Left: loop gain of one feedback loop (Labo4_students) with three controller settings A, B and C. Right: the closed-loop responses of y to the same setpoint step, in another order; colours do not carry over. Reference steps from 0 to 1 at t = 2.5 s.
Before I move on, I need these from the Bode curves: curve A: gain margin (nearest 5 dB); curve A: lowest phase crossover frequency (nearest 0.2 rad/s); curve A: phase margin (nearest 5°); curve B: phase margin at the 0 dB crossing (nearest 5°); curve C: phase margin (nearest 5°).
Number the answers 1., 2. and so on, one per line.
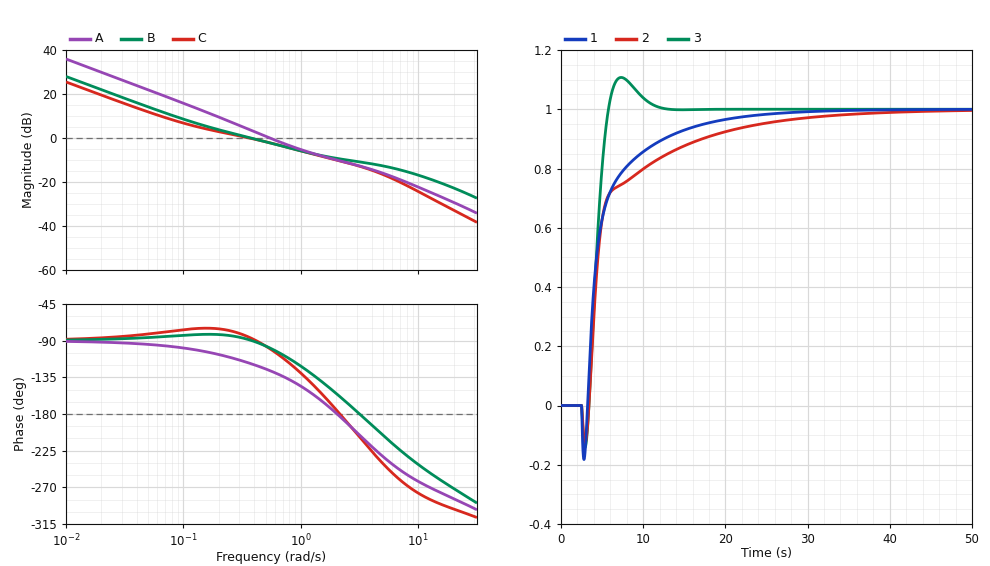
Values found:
1. 10 dB
2. 2.0 rad/s
3. 55°
4. 90°
5. 95°
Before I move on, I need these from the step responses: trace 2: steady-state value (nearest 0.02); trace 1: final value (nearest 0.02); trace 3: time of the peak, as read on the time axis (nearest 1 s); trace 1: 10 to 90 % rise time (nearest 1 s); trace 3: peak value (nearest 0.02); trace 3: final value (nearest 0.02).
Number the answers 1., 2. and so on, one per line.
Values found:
1. 1.00
2. 1.00
3. 7 s
4. 9 s
5. 1.10
6. 1.00
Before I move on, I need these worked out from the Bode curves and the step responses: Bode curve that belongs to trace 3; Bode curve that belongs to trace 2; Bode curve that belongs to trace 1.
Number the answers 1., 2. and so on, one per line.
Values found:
1. A
2. C
3. B
